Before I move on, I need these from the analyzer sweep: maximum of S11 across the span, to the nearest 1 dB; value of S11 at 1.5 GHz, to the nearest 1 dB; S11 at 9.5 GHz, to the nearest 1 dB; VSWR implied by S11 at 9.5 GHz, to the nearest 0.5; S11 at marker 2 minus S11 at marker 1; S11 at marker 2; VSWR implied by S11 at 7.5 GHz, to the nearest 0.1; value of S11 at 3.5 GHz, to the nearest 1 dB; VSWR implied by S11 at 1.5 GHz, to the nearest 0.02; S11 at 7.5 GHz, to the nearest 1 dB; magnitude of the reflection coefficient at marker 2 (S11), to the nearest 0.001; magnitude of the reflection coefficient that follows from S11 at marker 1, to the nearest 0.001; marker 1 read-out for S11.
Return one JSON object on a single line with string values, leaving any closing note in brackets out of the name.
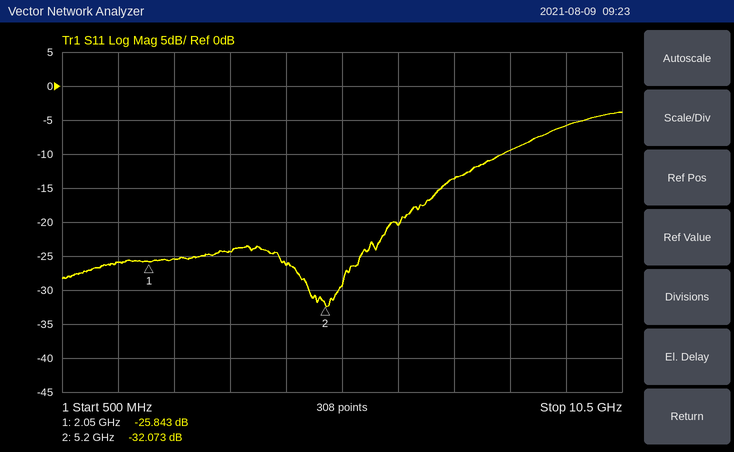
{"maximum of S11 across the span, to the nearest 1 dB": "-4 dB", "value of S11 at 1.5 GHz, to the nearest 1 dB": "-26 dB", "S11 at 9.5 GHz, to the nearest 1 dB": "-6 dB", "VSWR implied by S11 at 9.5 GHz, to the nearest 0.5": "3.0", "S11 at marker 2 minus S11 at marker 1": "-6.230 dB", "S11 at marker 2": "-32.073 dB", "VSWR implied by S11 at 7.5 GHz, to the nearest 0.1": "1.5", "value of S11 at 3.5 GHz, to the nearest 1 dB": "-24 dB", "VSWR implied by S11 at 1.5 GHz, to the nearest 0.02": "1.10", "S11 at 7.5 GHz, to the nearest 1 dB": "-14 dB", "magnitude of the reflection coefficient at marker 2 (S11), to the nearest 0.001": "0.025", "magnitude of the reflection coefficient that follows from S11 at marker 1, to the nearest 0.001": "0.051", "marker 1 read-out for S11": "-25.843 dB"}
